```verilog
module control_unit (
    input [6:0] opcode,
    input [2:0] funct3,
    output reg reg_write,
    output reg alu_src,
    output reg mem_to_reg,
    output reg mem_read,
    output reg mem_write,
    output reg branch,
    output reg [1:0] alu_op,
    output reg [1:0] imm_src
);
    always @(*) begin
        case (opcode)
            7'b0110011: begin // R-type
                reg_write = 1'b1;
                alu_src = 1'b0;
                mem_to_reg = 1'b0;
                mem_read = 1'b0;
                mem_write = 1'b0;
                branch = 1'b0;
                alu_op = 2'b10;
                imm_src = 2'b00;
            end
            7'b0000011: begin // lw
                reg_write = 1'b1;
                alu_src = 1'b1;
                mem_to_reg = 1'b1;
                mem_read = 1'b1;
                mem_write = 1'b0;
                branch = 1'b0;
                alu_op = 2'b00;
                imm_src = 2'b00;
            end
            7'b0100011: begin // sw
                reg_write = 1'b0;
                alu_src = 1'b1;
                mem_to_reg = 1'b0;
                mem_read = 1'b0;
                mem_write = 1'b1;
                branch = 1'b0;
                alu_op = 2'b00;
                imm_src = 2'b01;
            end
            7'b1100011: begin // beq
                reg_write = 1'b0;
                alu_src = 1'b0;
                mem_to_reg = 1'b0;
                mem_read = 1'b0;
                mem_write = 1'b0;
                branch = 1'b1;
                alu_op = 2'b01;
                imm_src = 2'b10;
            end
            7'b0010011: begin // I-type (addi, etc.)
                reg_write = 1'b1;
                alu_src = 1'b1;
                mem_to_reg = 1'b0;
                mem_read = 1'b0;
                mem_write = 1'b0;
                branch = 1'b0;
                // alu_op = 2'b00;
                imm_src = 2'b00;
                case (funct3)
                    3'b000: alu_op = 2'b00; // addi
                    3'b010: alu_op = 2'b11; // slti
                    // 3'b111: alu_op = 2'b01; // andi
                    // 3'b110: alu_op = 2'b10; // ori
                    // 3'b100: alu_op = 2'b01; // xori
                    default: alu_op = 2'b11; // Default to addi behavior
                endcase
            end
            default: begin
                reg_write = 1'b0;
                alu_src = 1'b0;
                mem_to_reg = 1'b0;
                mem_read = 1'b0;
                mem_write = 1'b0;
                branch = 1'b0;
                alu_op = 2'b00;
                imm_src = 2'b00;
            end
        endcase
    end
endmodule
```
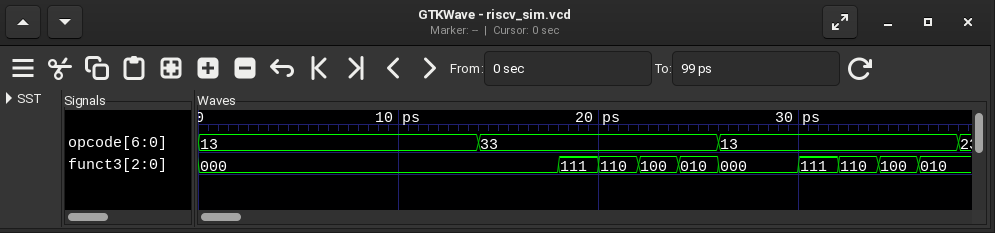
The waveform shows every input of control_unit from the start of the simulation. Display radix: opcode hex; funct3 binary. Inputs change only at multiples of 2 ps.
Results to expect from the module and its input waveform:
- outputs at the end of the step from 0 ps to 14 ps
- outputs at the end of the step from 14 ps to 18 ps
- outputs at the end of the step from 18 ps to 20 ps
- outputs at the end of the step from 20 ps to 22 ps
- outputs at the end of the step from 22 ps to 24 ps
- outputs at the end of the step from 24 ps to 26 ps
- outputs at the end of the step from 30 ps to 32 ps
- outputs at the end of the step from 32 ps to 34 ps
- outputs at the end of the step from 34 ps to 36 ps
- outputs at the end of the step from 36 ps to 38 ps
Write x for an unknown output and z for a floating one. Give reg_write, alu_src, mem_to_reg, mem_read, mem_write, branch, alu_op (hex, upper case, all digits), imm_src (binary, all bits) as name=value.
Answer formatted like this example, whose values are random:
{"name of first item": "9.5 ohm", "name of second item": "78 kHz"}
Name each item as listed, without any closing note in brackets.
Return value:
{"outputs at the end of the step from 0 ps to 14 ps": "reg_write=1, alu_src=1, mem_to_reg=0, mem_read=0, mem_write=0, branch=0, alu_op=0, imm_src=00", "outputs at the end of the step from 14 ps to 18 ps": "reg_write=1, alu_src=0, mem_to_reg=0, mem_read=0, mem_write=0, branch=0, alu_op=2, imm_src=00", "outputs at the end of the step from 18 ps to 20 ps": "reg_write=1, alu_src=0, mem_to_reg=0, mem_read=0, mem_write=0, branch=0, alu_op=2, imm_src=00", "outputs at the end of the step from 20 ps to 22 ps": "reg_write=1, alu_src=0, mem_to_reg=0, mem_read=0, mem_write=0, branch=0, alu_op=2, imm_src=00", "outputs at the end of the step from 22 ps to 24 ps": "reg_write=1, alu_src=0, mem_to_reg=0, mem_read=0, mem_write=0, branch=0, alu_op=2, imm_src=00", "outputs at the end of the step from 24 ps to 26 ps": "reg_write=1, alu_src=0, mem_to_reg=0, mem_read=0, mem_write=0, branch=0, alu_op=2, imm_src=00", "outputs at the end of the step from 30 ps to 32 ps": "reg_write=1, alu_src=1, mem_to_reg=0, mem_read=0, mem_write=0, branch=0, alu_op=3, imm_src=00", "outputs at the end of the step from 32 ps to 34 ps": "reg_write=1, alu_src=1, mem_to_reg=0, mem_read=0, mem_write=0, branch=0, alu_op=3, imm_src=00", "outputs at the end of the step from 34 ps to 36 ps": "reg_write=1, alu_src=1, mem_to_reg=0, mem_read=0, mem_write=0, branch=0, alu_op=3, imm_src=00", "outputs at the end of the step from 36 ps to 38 ps": "reg_write=1, alu_src=1, mem_to_reg=0, mem_read=0, mem_write=0, branch=0, alu_op=3, imm_src=00"}
